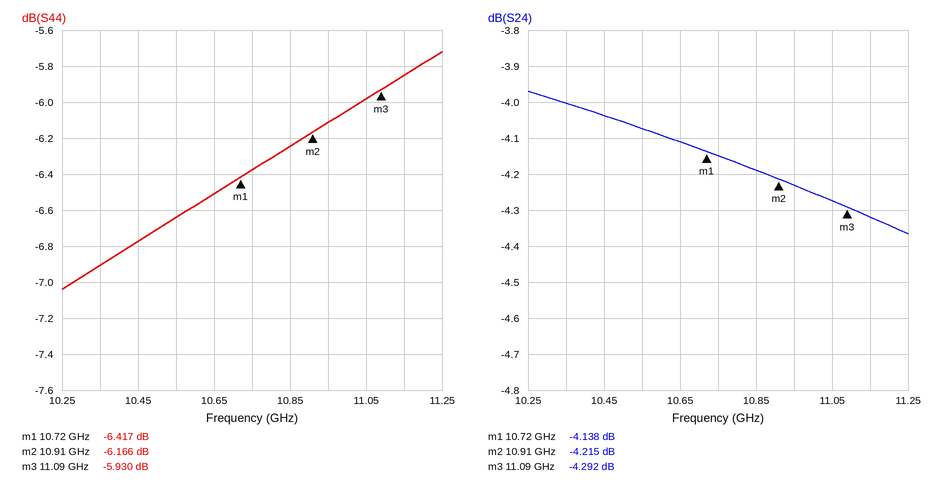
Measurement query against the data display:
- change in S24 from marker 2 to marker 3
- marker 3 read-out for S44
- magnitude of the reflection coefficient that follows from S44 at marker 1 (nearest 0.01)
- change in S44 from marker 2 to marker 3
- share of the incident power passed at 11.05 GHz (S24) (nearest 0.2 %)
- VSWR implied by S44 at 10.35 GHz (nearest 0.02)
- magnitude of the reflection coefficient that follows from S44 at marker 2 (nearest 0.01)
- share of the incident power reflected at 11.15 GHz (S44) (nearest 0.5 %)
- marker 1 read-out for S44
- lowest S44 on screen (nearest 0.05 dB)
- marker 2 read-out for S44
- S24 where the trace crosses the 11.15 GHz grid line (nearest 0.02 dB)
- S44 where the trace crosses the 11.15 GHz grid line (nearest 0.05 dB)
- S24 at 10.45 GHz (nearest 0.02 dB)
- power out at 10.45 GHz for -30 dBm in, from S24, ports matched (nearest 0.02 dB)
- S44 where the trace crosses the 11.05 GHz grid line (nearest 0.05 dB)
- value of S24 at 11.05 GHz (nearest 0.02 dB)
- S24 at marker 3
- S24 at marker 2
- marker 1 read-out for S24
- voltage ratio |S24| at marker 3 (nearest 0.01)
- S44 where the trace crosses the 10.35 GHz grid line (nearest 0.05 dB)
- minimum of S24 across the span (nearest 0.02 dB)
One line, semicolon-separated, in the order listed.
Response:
-0.077 dB; -5.930 dB; 0.48; 0.236 dB; 37.4 %; 2.64; 0.49; 26.0 %; -6.417 dB; -7.05 dB; -6.166 dB; -4.32 dB; -5.85 dB; -4.04 dB; -34.04 dBm; -6.00 dB; -4.28 dB; -4.292 dB; -4.215 dB; -4.138 dB; 0.61; -6.90 dB; -4.36 dB
